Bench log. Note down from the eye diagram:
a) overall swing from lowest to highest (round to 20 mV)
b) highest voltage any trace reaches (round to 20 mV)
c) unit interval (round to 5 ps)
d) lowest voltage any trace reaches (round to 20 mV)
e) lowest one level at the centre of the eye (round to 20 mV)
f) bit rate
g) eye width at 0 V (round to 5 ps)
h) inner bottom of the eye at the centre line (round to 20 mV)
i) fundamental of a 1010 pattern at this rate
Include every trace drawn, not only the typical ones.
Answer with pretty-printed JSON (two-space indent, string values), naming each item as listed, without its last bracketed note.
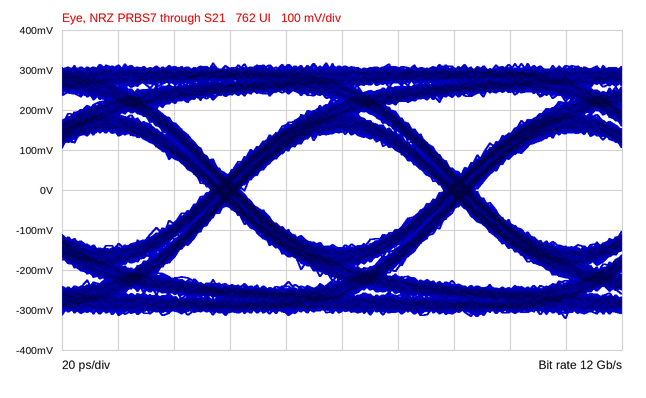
{
  "overall swing from lowest to highest": "640 mV",
  "highest voltage any trace reaches": "320 mV",
  "unit interval": "85 ps",
  "lowest voltage any trace reaches": "-320 mV",
  "lowest one level at the centre of the eye": "140 mV",
  "bit rate": "12 Gb/s",
  "eye width at 0 V": "70 ps",
  "inner bottom of the eye at the centre line": "-140 mV",
  "fundamental of a 1010 pattern at this rate": "6 GHz"
}
